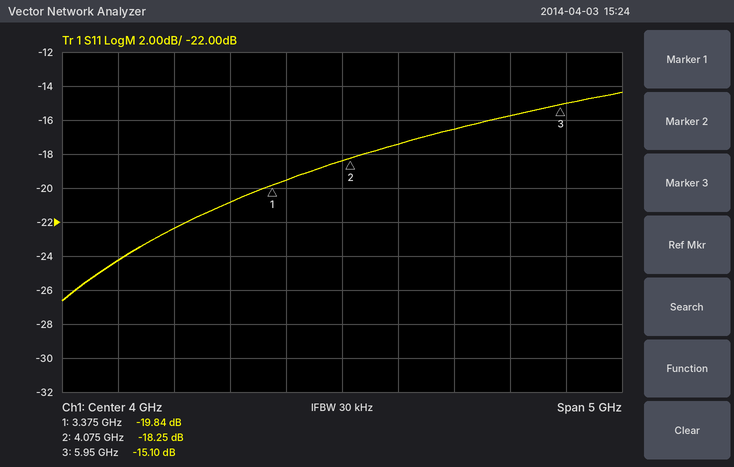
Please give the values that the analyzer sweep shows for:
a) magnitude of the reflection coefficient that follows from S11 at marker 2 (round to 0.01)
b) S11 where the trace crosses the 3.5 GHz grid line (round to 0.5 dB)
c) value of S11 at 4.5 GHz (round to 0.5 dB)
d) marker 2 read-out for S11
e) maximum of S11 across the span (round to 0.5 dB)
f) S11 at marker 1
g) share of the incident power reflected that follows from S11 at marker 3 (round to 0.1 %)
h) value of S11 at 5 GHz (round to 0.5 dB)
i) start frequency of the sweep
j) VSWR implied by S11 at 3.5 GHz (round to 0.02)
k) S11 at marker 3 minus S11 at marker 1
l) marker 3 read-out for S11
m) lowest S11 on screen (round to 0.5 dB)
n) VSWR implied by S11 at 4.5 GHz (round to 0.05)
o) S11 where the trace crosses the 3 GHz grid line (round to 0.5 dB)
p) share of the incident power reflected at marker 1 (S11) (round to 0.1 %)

0.12
-19.5 dB
-17.5 dB
-18.25 dB
-14.5 dB
-19.84 dB
3.1 %
-16.5 dB
1.5 GHz
1.24
4.74 dB
-15.10 dB
-26.5 dB
1.30
-21.0 dB
1.0 %
